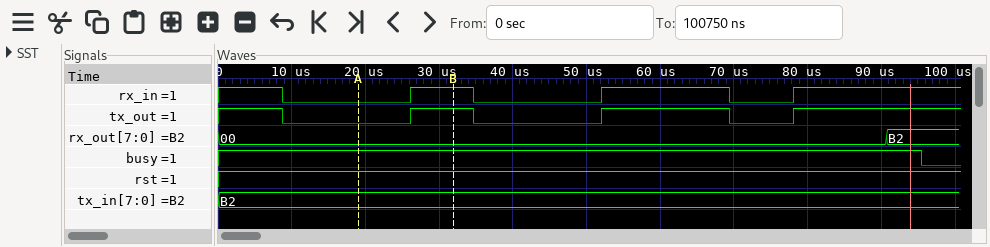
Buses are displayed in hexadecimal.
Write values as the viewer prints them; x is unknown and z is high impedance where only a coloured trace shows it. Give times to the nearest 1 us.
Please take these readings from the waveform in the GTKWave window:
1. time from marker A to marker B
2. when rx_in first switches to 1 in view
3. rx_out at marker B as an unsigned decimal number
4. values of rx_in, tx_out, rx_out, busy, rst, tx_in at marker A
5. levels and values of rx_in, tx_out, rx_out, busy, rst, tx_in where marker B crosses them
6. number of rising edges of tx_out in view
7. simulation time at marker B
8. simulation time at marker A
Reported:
13 us
26 us
0
rx_in=0, tx_out=0, rx_out=00, busy=1, rst=1, tx_in=B2
rx_in=1, tx_out=1, rx_out=00, busy=1, rst=1, tx_in=B2
3
32 us
19 us
